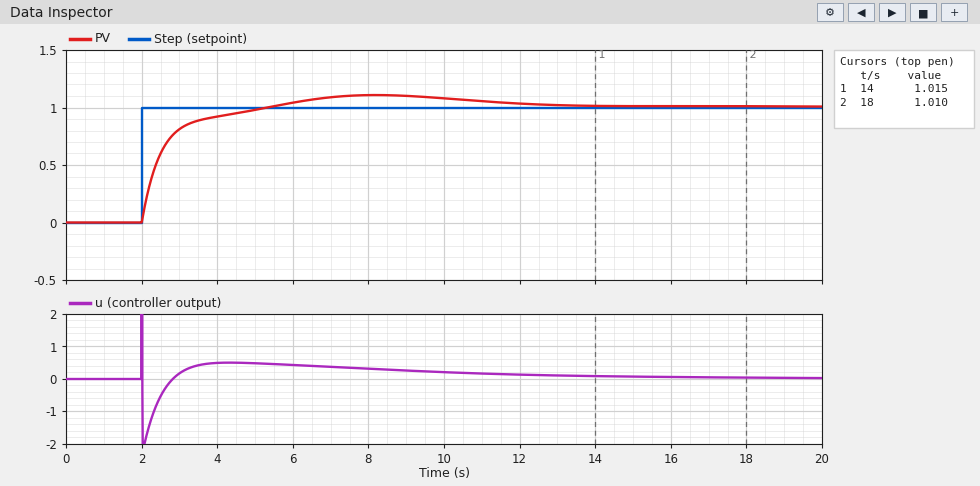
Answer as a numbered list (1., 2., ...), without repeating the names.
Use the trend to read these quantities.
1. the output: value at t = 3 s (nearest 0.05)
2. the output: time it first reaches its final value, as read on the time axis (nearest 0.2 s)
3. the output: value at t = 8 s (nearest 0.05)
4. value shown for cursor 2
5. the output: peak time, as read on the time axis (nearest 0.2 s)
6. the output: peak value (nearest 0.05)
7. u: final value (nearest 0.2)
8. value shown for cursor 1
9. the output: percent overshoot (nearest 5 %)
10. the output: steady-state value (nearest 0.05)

1. 0.80
2. 5.4 s
3. 1.10
4. 1.010
5. 8.2 s
6. 1.10
7. 0.0
8. 1.015
9. 10 %
10. 1.00
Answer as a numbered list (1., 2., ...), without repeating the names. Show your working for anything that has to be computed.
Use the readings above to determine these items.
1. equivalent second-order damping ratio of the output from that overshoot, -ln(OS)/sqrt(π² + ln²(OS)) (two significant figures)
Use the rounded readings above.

1. ln(0.1) = -2.303; 2.303 / sqrt(9.870 + 5.302) = 0.59
